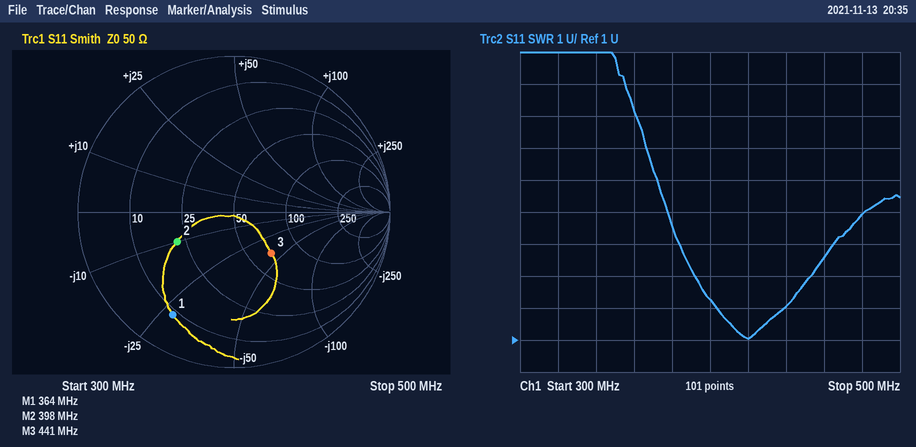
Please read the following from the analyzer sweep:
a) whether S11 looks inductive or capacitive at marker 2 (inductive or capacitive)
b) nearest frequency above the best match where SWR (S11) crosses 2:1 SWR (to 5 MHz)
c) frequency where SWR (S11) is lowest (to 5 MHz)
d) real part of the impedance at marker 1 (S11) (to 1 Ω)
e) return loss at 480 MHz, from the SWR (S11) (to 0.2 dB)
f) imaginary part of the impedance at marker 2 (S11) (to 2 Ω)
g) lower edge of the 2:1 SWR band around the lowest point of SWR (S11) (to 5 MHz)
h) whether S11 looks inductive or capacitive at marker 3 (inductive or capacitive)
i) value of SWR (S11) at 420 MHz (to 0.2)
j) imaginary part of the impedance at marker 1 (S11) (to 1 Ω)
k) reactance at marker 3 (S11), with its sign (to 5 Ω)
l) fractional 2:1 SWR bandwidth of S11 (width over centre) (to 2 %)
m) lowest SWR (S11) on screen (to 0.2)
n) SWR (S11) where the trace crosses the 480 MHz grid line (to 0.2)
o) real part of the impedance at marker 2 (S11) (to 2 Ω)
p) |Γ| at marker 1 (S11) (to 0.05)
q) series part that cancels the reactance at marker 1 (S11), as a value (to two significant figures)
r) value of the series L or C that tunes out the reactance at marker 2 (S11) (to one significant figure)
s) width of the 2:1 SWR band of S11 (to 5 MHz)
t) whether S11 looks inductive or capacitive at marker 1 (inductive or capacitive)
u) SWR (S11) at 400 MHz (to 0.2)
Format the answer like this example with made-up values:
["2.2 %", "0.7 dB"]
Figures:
["capacitive", "440 MHz", "420 MHz", "9 Ω", "3.6 dB", "-10 Ω", "405 MHz", "capacitive", "1.0", "-28 Ω", "-40 Ω", "8 %", "1.0", "5.0", "22 Ω", "0.75", "12 nH", "4 nH", "35 MHz", "capacitive", "2.2"]
